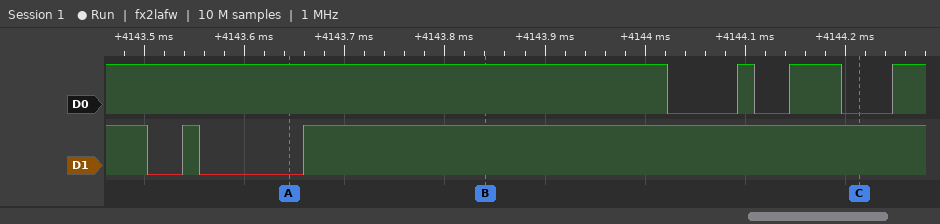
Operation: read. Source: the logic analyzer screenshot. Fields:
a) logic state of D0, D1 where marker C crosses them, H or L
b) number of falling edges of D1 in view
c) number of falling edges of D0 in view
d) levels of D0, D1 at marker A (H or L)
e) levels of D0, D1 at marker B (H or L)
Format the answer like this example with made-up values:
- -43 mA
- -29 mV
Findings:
- D0=L, D1=H
- 2
- 3
- D0=H, D1=L
- D0=H, D1=H
